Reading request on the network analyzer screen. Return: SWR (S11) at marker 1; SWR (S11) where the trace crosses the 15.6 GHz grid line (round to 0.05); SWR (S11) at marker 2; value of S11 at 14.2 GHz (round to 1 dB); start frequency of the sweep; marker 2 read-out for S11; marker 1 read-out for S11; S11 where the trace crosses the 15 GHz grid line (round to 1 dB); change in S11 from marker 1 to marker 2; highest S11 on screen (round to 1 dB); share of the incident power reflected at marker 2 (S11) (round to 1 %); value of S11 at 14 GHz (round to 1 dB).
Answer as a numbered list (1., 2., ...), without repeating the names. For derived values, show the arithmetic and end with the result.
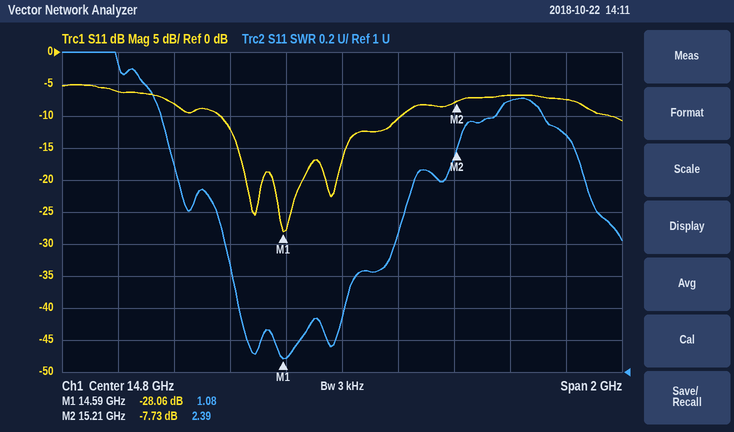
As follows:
1. 1.08
2. 2.50
3. 2.39
4. -8 dB
5. 13.8 GHz
6. -7.73 dB
7. -28.06 dB
8. -10 dB
9. -7.73 − (-28.06) = 20.33 dB
10. -5 dB
11. 10^(-7.73/10) ≈ 17 %
12. -6 dB
